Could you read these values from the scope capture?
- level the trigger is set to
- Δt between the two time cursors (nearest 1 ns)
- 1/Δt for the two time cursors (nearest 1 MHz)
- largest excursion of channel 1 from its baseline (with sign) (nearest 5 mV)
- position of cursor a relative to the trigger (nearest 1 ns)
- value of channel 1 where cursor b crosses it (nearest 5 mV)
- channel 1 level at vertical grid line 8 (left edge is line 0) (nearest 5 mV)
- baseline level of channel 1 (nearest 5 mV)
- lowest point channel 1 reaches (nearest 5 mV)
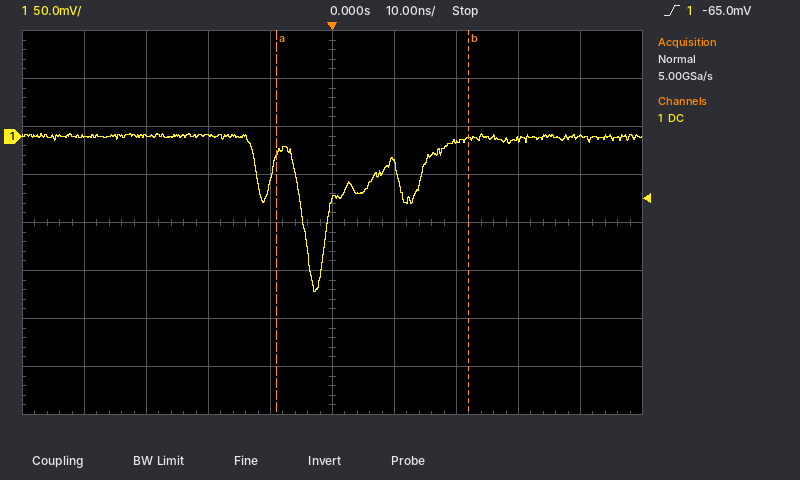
-65.0 mV
31 ns
32 MHz
-160 mV
-9 ns
-5 mV
-5 mV
0 mV
-160 mV
